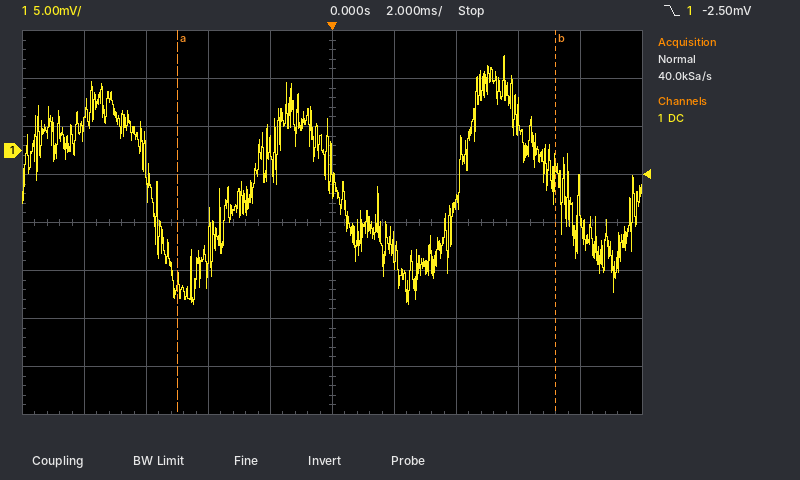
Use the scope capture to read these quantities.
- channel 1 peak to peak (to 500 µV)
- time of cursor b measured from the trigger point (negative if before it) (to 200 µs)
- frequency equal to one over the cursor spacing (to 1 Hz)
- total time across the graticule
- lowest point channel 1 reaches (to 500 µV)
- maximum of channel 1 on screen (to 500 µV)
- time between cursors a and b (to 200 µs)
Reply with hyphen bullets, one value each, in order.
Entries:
- 26.0 mV
- +7.2 ms
- 82 Hz
- 20 ms
- -16.0 mV
- 10.0 mV
- 12.2 ms
